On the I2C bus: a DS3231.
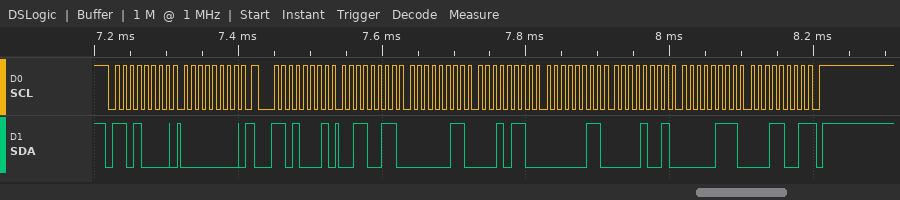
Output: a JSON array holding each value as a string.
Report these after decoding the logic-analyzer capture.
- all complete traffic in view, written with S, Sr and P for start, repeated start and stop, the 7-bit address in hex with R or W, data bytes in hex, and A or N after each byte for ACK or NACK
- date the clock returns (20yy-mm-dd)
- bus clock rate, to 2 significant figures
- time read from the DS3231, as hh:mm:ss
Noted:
["S 68W A 00 A Sr 68R A 33 A 03 A 16 A 03 A 09 A 07 A 19 N P", "2019-07-09", "100 kHz", "16:03:33"]
